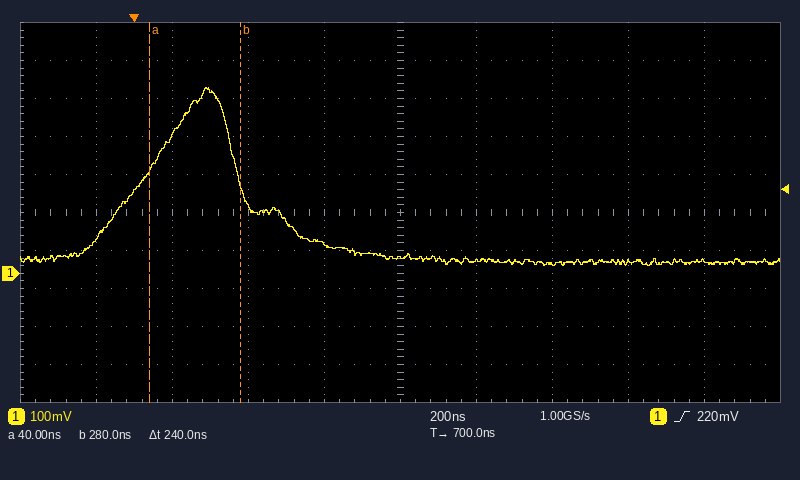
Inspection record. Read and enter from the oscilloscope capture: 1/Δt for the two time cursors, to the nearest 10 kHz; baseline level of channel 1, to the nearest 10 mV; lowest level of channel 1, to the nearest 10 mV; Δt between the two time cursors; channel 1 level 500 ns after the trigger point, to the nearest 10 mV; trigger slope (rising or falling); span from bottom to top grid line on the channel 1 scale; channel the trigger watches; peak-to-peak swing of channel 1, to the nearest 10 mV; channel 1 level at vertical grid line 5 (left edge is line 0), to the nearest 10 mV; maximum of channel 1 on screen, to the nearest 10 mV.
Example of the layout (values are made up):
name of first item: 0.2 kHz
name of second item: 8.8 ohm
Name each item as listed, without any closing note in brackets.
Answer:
1/Δt for the two time cursors, to the nearest 10 kHz: 4.17 MHz
baseline level of channel 1, to the nearest 10 mV: 30 mV
lowest level of channel 1, to the nearest 10 mV: 20 mV
Δt between the two time cursors: 240 ns
channel 1 level 500 ns after the trigger point, to the nearest 10 mV: 80 mV
trigger slope: rising
span from bottom to top grid line on the channel 1 scale: 1 V
channel the trigger watches: channel 1
peak-to-peak swing of channel 1, to the nearest 10 mV: 470 mV
channel 1 level at vertical grid line 5 (left edge is line 0), to the nearest 10 mV: 40 mV
maximum of channel 1 on screen, to the nearest 10 mV: 490 mV
